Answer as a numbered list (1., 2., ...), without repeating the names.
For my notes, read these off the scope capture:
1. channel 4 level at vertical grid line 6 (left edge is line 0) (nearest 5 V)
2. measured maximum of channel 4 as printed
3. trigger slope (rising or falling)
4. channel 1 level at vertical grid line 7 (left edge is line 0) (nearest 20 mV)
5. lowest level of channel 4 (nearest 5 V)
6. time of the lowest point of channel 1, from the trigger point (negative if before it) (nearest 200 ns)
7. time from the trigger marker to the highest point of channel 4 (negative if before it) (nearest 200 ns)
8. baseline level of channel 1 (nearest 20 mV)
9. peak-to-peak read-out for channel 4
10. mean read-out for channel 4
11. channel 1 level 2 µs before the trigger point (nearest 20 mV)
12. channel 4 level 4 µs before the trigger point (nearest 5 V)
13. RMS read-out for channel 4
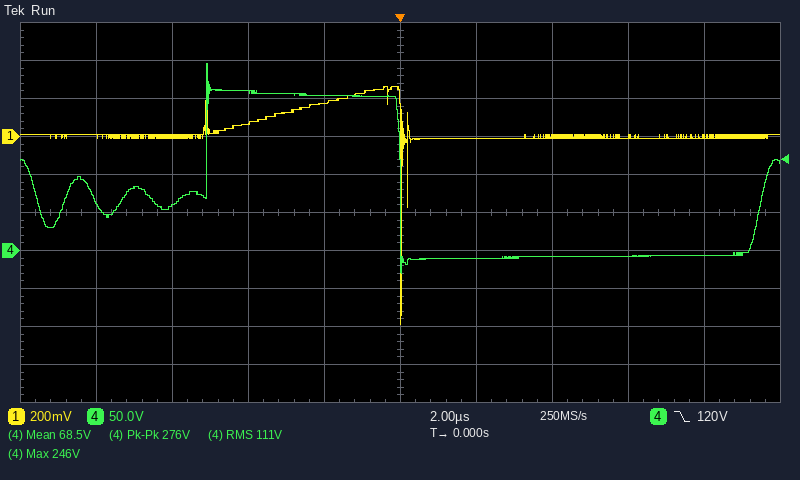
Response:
1. -10 V
2. 246 V
3. falling
4. 0 mV
5. -30 V
6. 0.0 µs
7. -5.0 µs
8. 0 mV
9. 276 V
10. 68.5 V
11. 180 mV
12. 210 V
13. 111 V
